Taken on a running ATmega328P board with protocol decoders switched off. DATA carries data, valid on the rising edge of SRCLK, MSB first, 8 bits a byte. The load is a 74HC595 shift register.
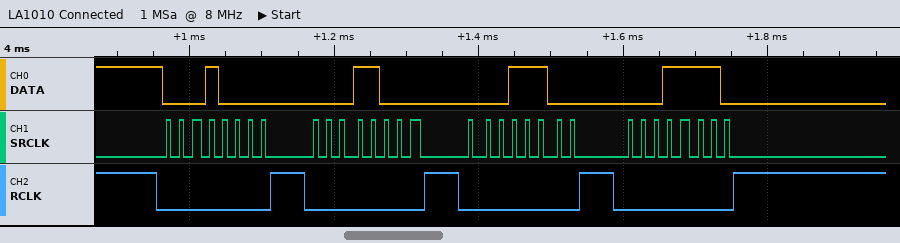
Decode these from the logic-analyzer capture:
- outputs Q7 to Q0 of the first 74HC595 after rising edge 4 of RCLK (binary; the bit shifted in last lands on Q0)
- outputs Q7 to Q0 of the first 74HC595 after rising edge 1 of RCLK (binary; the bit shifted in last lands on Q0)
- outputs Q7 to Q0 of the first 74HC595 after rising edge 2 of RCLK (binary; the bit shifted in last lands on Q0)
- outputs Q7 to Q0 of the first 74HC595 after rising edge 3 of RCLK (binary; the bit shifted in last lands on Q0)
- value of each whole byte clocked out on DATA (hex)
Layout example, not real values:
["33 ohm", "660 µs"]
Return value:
["00011110", "00010000", "00011000", "00011100", "10 18 1C 1E"]
